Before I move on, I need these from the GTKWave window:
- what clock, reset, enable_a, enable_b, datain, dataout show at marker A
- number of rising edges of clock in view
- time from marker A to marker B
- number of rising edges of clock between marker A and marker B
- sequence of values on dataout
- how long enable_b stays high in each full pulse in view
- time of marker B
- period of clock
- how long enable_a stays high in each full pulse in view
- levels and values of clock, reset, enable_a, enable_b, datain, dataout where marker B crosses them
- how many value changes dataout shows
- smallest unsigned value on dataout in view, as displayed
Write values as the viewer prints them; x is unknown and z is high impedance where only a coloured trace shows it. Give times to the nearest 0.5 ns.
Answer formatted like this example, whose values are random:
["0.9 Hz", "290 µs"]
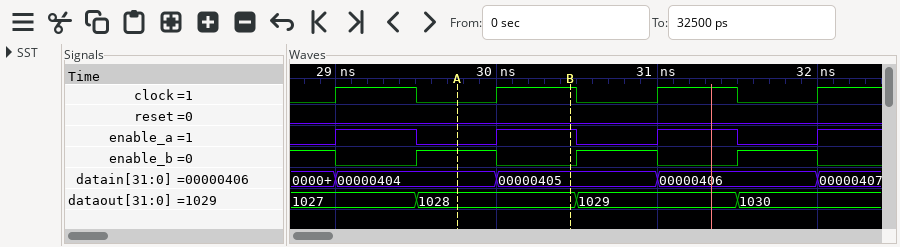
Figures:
["clock=0, reset=0, enable_a=0, enable_b=1, datain=00000404, dataout=1028", "4", "0.5 ns", "1", "1027, 1028, 1029, 1030", "0.5 ns, 0.5 ns, 0.5 ns", "30.5 ns", "1 ns", "0.5 ns, 0.5 ns, 0.5 ns", "clock=1, reset=0, enable_a=1, enable_b=0, datain=00000405, dataout=1028", "3", "1027"]
